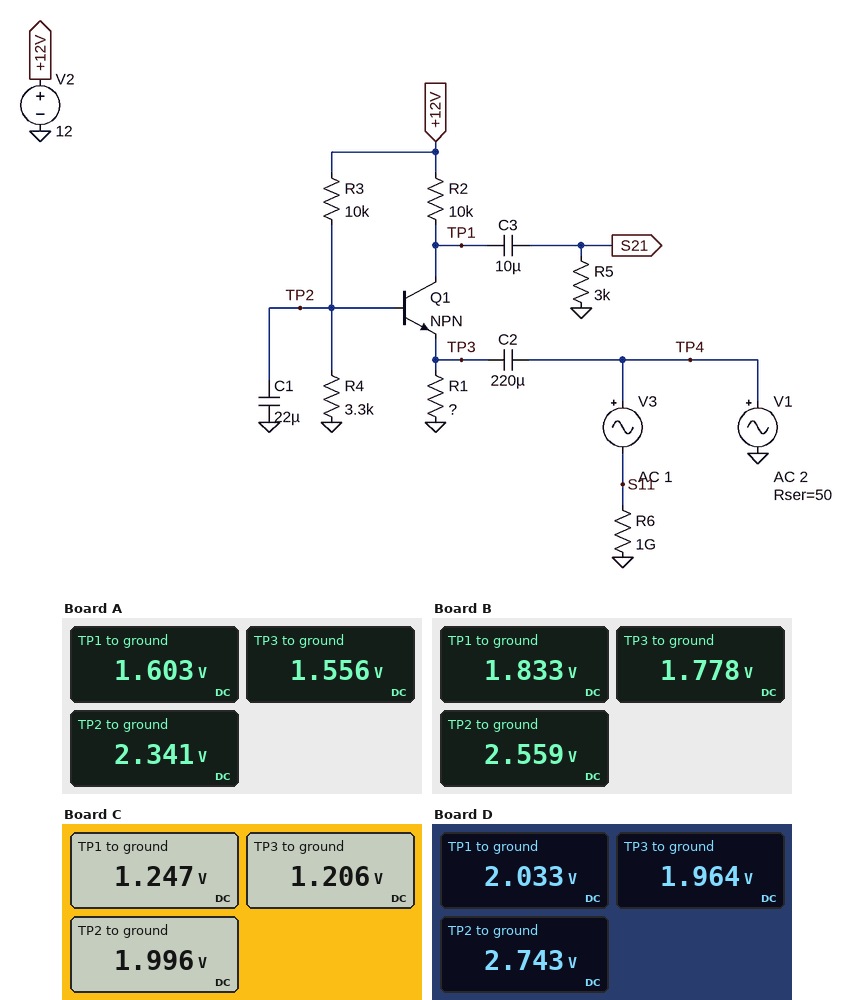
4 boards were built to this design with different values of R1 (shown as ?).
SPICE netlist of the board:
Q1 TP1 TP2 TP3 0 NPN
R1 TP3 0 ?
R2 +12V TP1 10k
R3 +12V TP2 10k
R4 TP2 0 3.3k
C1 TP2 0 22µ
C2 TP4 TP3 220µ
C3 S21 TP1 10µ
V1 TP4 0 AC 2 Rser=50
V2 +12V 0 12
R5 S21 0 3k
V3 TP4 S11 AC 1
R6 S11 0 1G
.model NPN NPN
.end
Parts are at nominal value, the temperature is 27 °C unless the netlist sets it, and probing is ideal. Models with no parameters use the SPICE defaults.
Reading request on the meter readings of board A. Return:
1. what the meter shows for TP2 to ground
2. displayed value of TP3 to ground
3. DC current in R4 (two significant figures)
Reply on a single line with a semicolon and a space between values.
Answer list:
2.341 V; 1.556 V; 710 µA
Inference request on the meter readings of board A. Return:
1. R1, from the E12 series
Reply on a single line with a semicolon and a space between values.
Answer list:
1.2 kΩ
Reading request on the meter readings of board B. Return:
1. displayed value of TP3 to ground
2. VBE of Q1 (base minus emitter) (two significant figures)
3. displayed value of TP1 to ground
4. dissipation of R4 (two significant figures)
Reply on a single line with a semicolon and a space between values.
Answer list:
1.778 V; 780 mV; 1.833 V; 2.0 mW
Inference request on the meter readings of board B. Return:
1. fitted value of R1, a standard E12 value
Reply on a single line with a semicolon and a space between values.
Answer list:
1.5 kΩ
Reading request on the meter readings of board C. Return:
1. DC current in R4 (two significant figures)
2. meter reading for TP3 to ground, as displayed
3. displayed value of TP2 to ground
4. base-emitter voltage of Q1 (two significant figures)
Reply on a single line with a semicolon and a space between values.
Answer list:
600 µA; 1.206 V; 1.996 V; 790 mV
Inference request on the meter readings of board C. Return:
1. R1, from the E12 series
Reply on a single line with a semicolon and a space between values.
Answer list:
820 Ω
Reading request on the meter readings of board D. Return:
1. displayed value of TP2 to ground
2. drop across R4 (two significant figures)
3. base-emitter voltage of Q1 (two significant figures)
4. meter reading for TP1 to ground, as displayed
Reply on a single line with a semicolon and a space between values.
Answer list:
2.743 V; 2.7 V; 780 mV; 2.033 V
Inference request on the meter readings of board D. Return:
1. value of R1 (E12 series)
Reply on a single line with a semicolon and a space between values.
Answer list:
1.8 kΩ
